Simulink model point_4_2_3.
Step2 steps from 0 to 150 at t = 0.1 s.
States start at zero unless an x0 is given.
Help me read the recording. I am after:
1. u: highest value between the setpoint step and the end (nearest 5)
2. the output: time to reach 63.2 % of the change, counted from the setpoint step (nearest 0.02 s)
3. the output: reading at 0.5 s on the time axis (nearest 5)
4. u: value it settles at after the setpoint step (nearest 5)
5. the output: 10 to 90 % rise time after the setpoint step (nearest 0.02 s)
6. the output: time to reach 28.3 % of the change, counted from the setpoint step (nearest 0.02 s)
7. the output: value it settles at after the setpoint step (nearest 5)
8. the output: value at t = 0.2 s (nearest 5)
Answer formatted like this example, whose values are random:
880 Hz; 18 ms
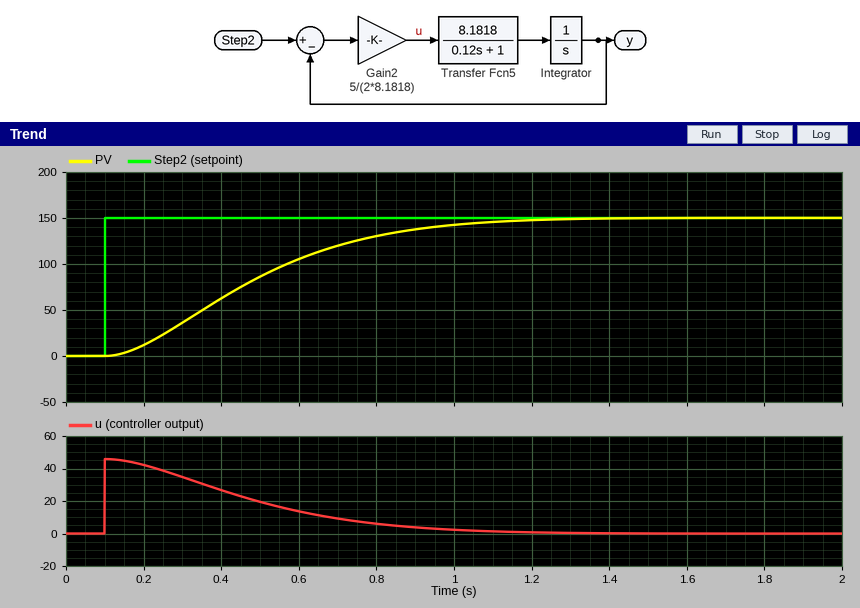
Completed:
45; 0.44 s; 85; 0; 0.64 s; 0.22 s; 150; 10
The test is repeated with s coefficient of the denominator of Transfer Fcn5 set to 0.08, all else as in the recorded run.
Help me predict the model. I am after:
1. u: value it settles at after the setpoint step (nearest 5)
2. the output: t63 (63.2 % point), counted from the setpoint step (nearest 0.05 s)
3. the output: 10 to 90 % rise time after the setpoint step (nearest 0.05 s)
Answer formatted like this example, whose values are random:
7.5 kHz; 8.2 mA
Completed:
0; 0.40 s; 0.70 s
